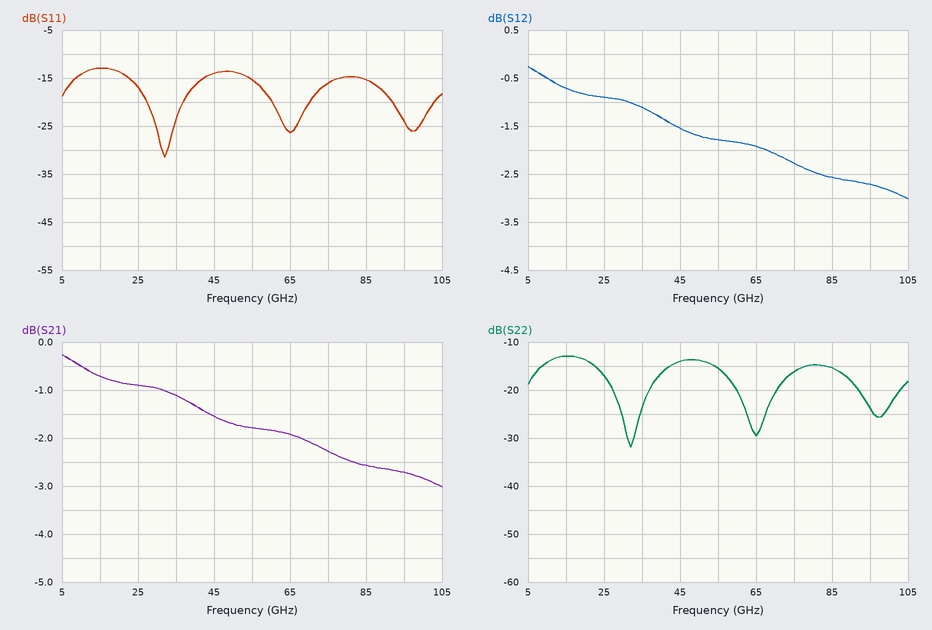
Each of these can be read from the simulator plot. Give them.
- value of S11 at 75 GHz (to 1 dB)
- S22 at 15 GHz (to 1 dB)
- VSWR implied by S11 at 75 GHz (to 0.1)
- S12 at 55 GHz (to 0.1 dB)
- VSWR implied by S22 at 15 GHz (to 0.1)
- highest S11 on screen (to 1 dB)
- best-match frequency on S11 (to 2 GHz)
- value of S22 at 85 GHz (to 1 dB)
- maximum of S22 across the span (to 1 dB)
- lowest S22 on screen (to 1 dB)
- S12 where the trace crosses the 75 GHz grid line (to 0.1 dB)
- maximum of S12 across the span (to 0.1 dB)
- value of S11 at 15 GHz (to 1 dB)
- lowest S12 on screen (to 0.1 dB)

-16 dB
-13 dB
1.4
-1.8 dB
1.6
-13 dB
32 GHz
-15 dB
-13 dB
-32 dB
-2.3 dB
-0.3 dB
-13 dB
-3.0 dB
